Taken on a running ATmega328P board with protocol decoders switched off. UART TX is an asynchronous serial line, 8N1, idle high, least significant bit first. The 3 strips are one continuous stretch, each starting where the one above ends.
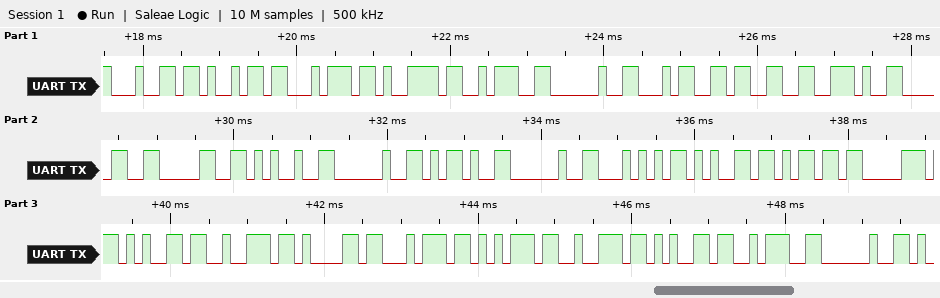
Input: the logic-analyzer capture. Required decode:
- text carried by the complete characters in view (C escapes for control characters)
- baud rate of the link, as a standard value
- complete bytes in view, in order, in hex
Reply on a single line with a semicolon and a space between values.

"dity: 43.00% - Temperature: "; 9600 baud; 64 69 74 79 3A 20 34 33 2E 30 30 25 20 2D 20 54 65 6D 70 65 72 61 74 75 72 65 3A 20
